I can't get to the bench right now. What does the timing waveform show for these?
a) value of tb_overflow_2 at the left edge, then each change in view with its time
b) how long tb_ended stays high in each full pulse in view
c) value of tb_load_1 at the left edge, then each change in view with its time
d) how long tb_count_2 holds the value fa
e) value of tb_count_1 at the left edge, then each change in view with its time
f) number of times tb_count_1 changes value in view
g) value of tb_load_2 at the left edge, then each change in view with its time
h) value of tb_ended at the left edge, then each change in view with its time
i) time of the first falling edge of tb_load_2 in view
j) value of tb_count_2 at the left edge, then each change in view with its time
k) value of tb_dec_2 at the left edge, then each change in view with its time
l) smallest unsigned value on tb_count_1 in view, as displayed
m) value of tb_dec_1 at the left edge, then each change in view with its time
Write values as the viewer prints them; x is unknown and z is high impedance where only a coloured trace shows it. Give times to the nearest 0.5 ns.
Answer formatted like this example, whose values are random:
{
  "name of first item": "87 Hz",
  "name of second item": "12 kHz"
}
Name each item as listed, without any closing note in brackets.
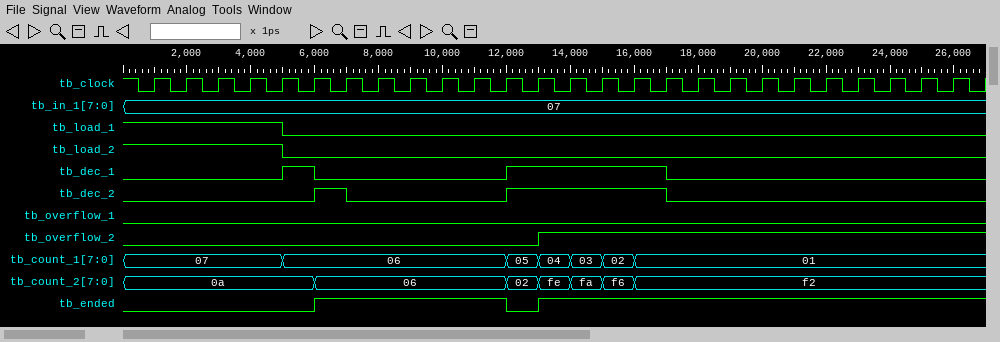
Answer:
{
  "value of tb_overflow_2 at the left edge, then each change in view with its time": "0, 1 at 13 ns",
  "how long tb_ended stays high in each full pulse in view": "6 ns",
  "value of tb_load_1 at the left edge, then each change in view with its time": "1, 0 at 5 ns",
  "how long tb_count_2 holds the value fa": "1 ns",
  "value of tb_count_1 at the left edge, then each change in view with its time": "07, 06 at 5 ns, 05 at 12 ns, 04 at 13 ns, 03 at 14 ns, 02 at 15 ns, 01 at 16 ns",
  "number of times tb_count_1 changes value in view": "6",
  "value of tb_load_2 at the left edge, then each change in view with its time": "1, 0 at 5 ns",
  "value of tb_ended at the left edge, then each change in view with its time": "0, 1 at 6 ns, 0 at 12 ns, 1 at 13 ns",
  "time of the first falling edge of tb_load_2 in view": "5 ns",
  "value of tb_count_2 at the left edge, then each change in view with its time": "0a, 06 at 6 ns, 02 at 12 ns, fe at 13 ns, fa at 14 ns, f6 at 15 ns, f2 at 16 ns",
  "value of tb_dec_2 at the left edge, then each change in view with its time": "0, 1 at 6 ns, 0 at 7 ns, 1 at 12 ns, 0 at 17 ns",
  "smallest unsigned value on tb_count_1 in view, as displayed": "01",
  "value of tb_dec_1 at the left edge, then each change in view with its time": "0, 1 at 5 ns, 0 at 6 ns, 1 at 12 ns, 0 at 17 ns"
}
